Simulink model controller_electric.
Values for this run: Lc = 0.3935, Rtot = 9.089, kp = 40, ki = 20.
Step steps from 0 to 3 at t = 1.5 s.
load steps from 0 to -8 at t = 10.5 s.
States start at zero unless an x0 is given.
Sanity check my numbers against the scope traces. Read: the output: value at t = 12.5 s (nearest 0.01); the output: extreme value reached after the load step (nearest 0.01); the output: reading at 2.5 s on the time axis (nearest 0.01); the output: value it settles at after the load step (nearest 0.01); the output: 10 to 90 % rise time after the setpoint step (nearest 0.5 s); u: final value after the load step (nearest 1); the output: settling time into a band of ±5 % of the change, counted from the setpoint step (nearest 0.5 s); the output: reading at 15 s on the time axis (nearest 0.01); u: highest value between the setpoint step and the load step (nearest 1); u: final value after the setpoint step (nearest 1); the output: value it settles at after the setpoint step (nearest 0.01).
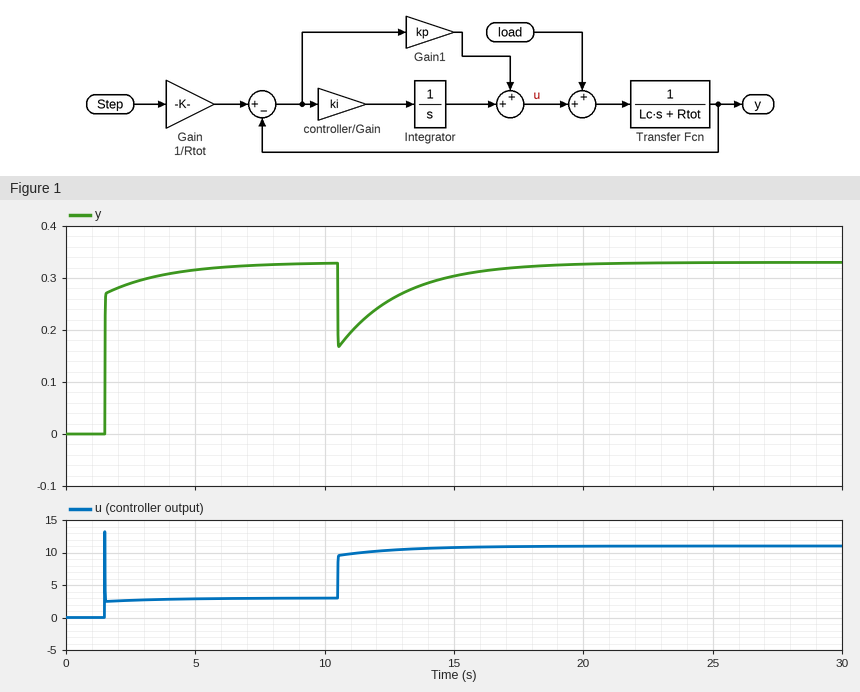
0.26
0.17
0.29
0.33
1.5 s
11
3.0 s
0.30
13
3
0.33
